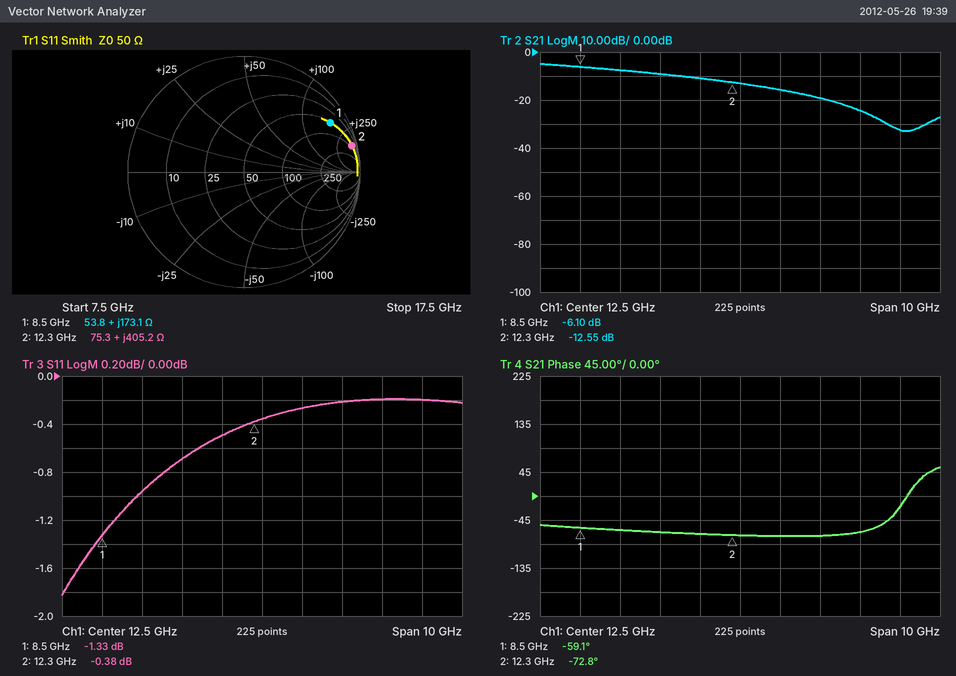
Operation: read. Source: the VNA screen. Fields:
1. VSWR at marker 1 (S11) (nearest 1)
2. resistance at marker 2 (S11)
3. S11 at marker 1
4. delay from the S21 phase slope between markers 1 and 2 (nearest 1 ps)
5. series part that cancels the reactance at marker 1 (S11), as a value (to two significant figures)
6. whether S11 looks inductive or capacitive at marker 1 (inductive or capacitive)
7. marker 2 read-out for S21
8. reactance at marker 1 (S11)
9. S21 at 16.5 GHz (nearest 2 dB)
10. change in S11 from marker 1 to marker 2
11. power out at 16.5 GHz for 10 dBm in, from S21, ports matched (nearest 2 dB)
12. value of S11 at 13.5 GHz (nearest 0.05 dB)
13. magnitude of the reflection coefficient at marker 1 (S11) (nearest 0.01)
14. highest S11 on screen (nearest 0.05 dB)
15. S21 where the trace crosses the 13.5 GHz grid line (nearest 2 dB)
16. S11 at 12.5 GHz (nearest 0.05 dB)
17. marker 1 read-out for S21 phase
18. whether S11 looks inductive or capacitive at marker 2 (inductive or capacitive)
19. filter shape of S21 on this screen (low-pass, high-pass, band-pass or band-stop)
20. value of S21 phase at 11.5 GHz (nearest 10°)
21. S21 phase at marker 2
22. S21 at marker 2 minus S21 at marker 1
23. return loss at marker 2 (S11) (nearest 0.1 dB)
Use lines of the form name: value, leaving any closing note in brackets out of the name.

VSWR at marker 1 (S11): 13
resistance at marker 2: 75.3 Ω
S11 at marker 1: -1.33 dB
delay from the S21 phase slope between markers 1 and 2: 10 ps
series part that cancels the reactance at marker 1 (S11), as a value: 110 fF
whether S11 looks inductive or capacitive at marker 1: inductive
marker 2 read-out for S21: -12.55 dB
reactance at marker 1: +173.1 Ω
S21 at 16.5 GHz: -32 dB
change in S11 from marker 1 to marker 2: 0.95 dB
power out at 16.5 GHz for 10 dBm in, from S21, ports matched: -22 dBm
value of S11 at 13.5 GHz: -0.25 dB
magnitude of the reflection coefficient at marker 1 (S11): 0.86
highest S11 on screen: -0.20 dB
S21 where the trace crosses the 13.5 GHz grid line: -16 dB
S11 at 12.5 GHz: -0.35 dB
marker 1 read-out for S21 phase: -59.1°
whether S11 looks inductive or capacitive at marker 2: inductive
filter shape of S21 on this screen: low-pass
value of S21 phase at 11.5 GHz: -70°
S21 phase at marker 2: -72.8°
S21 at marker 2 minus S21 at marker 1: -6.45 dB
return loss at marker 2 (S11): 0.4 dB
